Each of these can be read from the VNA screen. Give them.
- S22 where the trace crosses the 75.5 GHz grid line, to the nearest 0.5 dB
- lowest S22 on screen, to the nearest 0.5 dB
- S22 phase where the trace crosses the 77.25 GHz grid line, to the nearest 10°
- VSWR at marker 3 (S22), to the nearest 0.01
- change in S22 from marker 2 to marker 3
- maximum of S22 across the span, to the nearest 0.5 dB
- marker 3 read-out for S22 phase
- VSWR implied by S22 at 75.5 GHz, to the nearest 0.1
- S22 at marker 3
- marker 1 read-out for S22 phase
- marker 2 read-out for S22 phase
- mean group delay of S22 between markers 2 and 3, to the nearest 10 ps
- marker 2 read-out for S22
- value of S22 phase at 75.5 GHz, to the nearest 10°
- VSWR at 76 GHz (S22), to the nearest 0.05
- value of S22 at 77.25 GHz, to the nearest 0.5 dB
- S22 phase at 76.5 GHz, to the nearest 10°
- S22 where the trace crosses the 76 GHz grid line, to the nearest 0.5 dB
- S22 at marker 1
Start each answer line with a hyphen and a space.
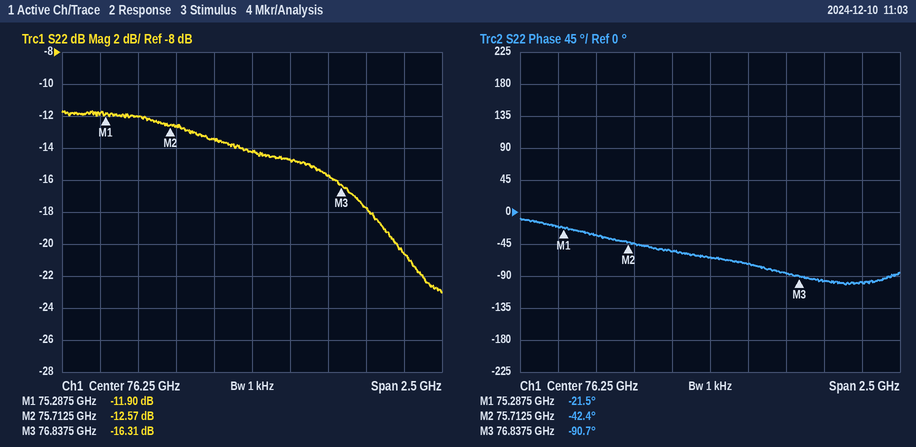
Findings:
- -12.0 dB
- -23.0 dB
- -100°
- 1.36
- -3.74 dB
- -11.5 dB
- -90.7°
- 1.7
- -16.31 dB
- -21.5°
- -42.4°
- 120 ps
- -12.57 dB
- -30°
- 1.55
- -20.5 dB
- -70°
- -13.5 dB
- -11.90 dB
